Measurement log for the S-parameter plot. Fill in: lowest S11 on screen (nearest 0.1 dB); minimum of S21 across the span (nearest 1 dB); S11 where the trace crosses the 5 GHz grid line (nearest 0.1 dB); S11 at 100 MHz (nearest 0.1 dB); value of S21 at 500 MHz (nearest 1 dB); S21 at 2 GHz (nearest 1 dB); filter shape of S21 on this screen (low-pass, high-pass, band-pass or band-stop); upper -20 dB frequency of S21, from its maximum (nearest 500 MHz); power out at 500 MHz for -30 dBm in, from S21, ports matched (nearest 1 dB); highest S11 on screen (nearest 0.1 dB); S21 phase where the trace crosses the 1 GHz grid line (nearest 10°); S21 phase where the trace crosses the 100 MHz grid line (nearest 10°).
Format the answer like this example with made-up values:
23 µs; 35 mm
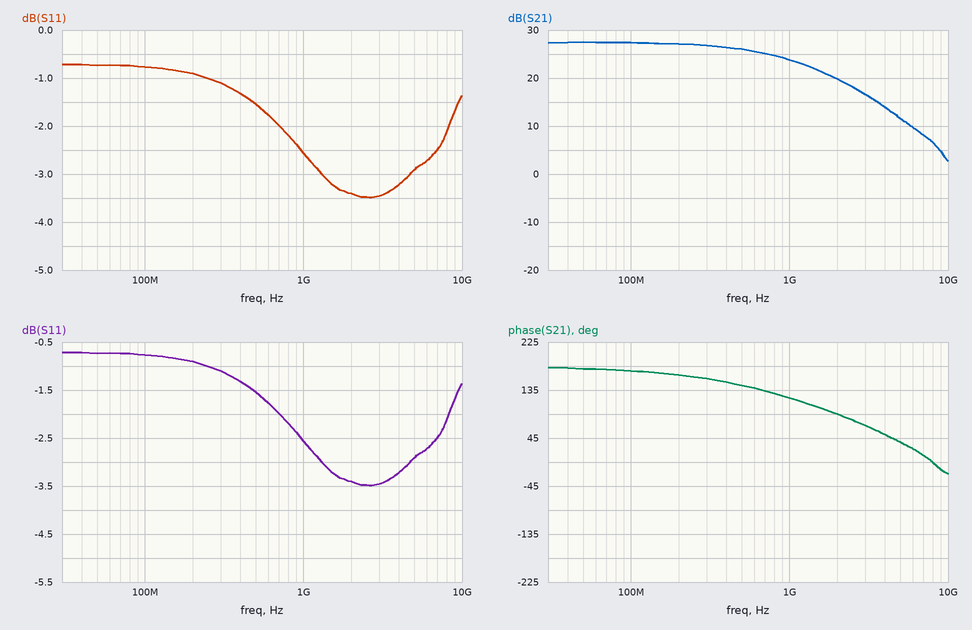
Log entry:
-3.5 dB; 3 dB; -2.9 dB; -0.8 dB; 26 dB; 20 dB; low-pass; 7.5 GHz; -4 dBm; -0.7 dB; 120°; 170°
